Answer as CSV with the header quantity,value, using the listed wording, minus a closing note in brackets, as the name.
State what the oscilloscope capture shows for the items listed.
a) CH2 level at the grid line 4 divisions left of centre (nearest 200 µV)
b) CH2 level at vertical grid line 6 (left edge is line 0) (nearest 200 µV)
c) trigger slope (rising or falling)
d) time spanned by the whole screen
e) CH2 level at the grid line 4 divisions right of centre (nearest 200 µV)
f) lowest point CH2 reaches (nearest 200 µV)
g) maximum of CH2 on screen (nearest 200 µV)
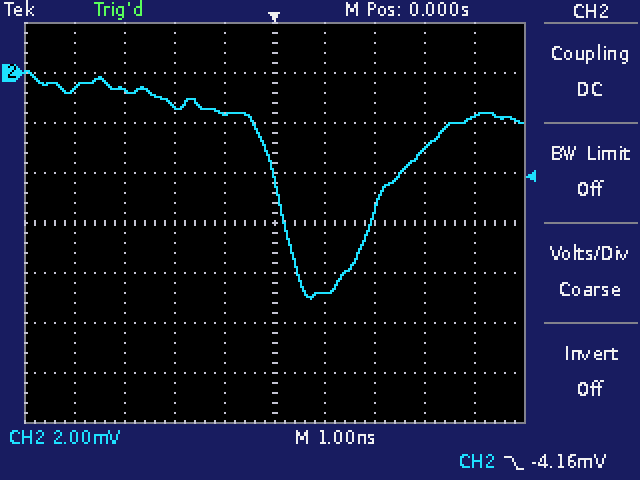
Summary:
quantity,value
CH2 level at the grid line 4 divisions left of centre,-600 µV
CH2 level at vertical grid line 6 (left edge is line 0),-8.8 mV
trigger slope,falling
time spanned by the whole screen,10 ns
CH2 level at the grid line 4 divisions right of centre,-1.8 mV
lowest point CH2 reaches,-9.0 mV
maximum of CH2 on screen,0.0 mV
